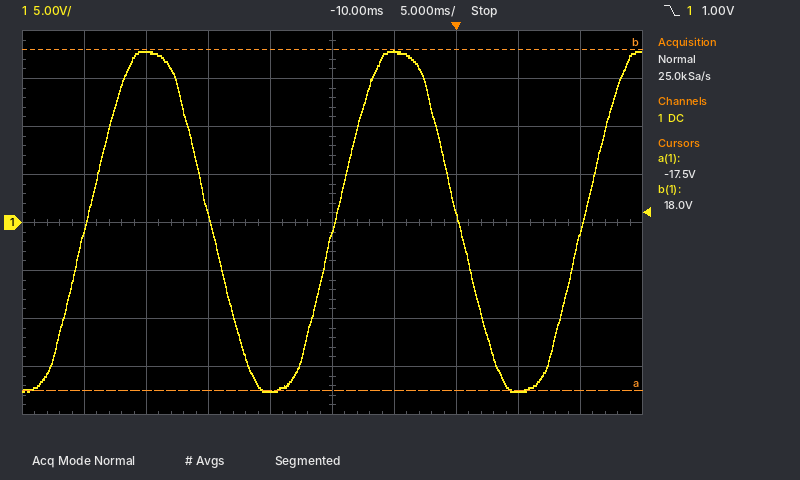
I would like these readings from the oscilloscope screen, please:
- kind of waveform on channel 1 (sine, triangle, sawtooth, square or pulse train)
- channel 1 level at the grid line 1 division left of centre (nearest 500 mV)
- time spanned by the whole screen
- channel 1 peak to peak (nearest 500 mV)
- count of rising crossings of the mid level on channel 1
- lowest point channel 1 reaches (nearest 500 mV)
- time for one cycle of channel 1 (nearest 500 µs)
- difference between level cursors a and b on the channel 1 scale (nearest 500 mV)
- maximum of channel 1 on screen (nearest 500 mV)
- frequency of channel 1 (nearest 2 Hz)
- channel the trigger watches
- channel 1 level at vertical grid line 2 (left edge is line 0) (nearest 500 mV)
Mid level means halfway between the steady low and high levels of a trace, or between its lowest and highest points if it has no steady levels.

sine
-17.5 V
50 ms
35.5 V
3
-17.5 V
20.0 ms
35.5 V
18.0 V
50 Hz
channel 1
18.0 V
